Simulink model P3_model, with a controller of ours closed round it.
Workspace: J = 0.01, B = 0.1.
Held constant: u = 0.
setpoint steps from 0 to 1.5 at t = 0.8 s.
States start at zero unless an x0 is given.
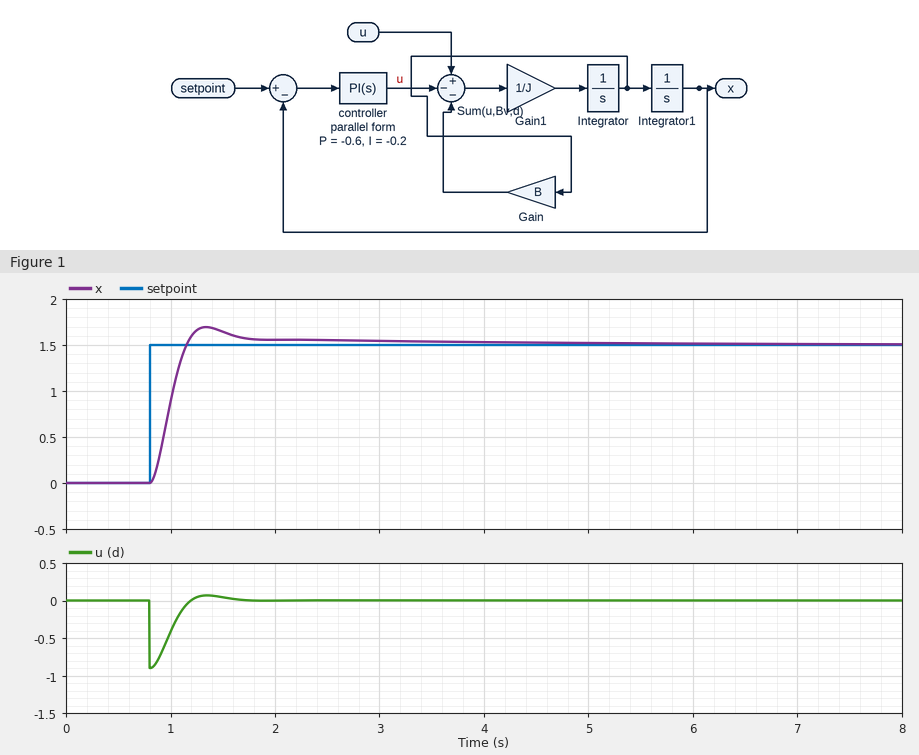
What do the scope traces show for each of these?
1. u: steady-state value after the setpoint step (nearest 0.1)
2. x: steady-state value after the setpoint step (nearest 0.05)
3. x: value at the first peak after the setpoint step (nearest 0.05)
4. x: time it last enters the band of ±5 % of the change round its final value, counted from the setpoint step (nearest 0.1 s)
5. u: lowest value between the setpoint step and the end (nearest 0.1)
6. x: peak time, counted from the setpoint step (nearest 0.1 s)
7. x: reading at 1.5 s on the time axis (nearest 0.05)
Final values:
0.0
1.50
1.70
0.9 s
-0.9
0.5 s
1.65
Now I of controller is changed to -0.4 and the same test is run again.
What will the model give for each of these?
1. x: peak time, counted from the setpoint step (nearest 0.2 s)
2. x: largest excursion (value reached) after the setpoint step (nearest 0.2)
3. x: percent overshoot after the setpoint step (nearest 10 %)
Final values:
0.6 s
1.8
20 %
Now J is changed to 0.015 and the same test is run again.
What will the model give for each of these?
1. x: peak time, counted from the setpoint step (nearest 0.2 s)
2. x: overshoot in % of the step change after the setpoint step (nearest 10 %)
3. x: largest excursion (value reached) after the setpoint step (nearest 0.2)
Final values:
0.6 s
20 %
1.8
